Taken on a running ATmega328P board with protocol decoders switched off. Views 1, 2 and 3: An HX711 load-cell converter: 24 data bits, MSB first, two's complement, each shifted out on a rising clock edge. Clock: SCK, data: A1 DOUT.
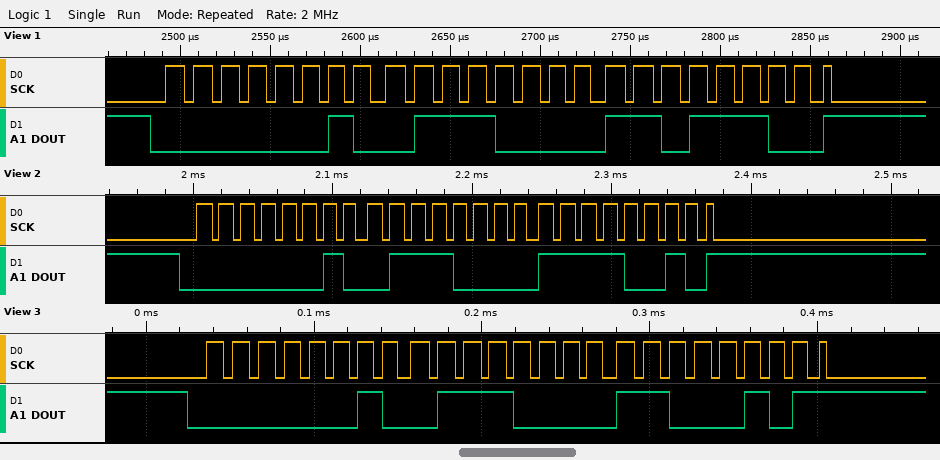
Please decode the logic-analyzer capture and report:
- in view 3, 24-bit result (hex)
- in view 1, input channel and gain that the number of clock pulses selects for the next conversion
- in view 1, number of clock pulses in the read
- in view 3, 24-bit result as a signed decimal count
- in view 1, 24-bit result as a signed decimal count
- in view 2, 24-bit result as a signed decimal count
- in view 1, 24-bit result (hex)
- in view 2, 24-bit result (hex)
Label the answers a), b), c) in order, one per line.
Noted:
a) 0x0270C5
b) channel A, gain 128
c) 25
d) 159941
e) 159964
f) 159986
g) 0x0270DC
h) 0x0270F2
